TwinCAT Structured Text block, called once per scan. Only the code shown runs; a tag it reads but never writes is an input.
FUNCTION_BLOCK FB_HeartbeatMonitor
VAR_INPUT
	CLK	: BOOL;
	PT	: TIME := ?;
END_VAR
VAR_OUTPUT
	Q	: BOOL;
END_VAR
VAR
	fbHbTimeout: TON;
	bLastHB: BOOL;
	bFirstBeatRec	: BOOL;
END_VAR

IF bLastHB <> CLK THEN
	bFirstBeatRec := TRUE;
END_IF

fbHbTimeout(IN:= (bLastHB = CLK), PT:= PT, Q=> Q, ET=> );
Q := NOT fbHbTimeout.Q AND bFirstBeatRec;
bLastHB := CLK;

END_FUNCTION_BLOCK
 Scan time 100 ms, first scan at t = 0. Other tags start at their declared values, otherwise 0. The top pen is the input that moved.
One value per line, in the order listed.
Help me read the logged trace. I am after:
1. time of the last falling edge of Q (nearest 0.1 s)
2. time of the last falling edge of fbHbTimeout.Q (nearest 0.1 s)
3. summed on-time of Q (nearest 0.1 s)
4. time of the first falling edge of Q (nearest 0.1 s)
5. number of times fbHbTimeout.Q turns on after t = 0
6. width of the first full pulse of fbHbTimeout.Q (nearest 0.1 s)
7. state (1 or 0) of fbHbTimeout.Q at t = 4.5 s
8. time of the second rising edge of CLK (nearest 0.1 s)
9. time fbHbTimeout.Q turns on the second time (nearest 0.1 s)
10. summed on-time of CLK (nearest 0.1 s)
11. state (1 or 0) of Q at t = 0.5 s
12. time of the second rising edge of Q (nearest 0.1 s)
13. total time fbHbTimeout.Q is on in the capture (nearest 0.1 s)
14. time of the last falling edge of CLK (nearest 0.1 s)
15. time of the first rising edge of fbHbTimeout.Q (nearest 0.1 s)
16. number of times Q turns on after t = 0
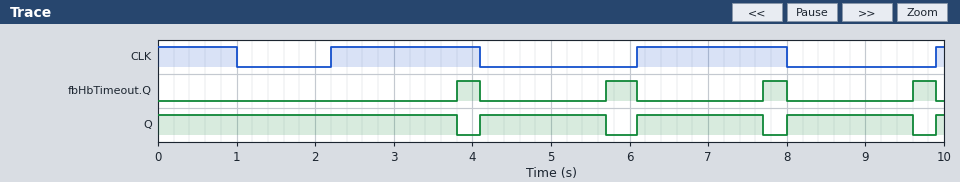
9.6 s
9.9 s
8.7 s
3.8 s
4
0.3 s
0
6.1 s
5.7 s
4.9 s
1
6.1 s
1.3 s
8.0 s
3.8 s
4
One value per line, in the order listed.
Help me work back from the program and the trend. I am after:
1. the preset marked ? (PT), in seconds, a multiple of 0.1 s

1.5 s
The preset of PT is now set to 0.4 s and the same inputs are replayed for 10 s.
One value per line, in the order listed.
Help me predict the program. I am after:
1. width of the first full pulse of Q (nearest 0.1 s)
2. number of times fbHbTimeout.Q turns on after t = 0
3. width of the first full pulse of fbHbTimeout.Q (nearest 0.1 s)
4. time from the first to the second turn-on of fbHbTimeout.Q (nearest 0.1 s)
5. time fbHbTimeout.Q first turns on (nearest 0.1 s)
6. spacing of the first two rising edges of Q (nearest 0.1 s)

0.5 s
6
0.5 s
1.0 s
0.5 s
1.2 s
